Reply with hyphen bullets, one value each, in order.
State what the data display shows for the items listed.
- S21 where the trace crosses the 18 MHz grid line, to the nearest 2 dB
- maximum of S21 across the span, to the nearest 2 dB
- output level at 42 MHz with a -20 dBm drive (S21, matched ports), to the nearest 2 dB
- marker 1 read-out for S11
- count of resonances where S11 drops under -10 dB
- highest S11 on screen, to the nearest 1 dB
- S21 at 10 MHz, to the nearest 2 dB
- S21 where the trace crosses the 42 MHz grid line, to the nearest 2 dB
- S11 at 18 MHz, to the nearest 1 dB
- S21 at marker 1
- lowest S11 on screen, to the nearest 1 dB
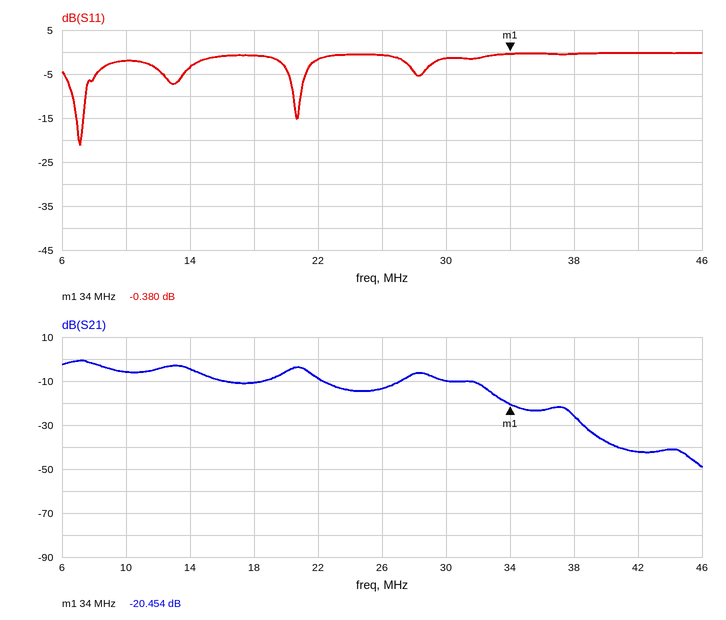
- -10 dB
- 0 dB
- -62 dBm
- -0.380 dB
- 2
- 0 dB
- -6 dB
- -42 dB
- -1 dB
- -20.454 dB
- -21 dB
